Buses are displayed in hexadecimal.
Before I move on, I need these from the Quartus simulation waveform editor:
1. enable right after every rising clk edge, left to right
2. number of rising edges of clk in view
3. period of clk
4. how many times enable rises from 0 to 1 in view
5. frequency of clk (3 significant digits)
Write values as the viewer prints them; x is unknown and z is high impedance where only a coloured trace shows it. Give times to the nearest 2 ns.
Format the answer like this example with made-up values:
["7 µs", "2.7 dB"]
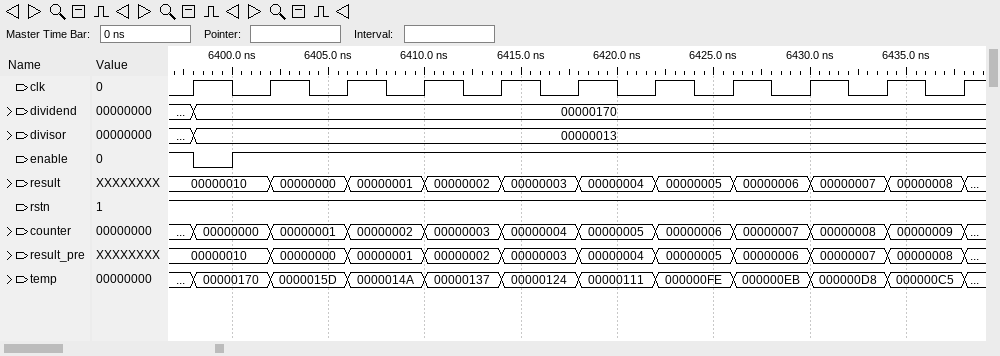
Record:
["0 1 1 1 1 1 1 1 1 1 1", "11", "4 ns", "1", "250 MHz"]
